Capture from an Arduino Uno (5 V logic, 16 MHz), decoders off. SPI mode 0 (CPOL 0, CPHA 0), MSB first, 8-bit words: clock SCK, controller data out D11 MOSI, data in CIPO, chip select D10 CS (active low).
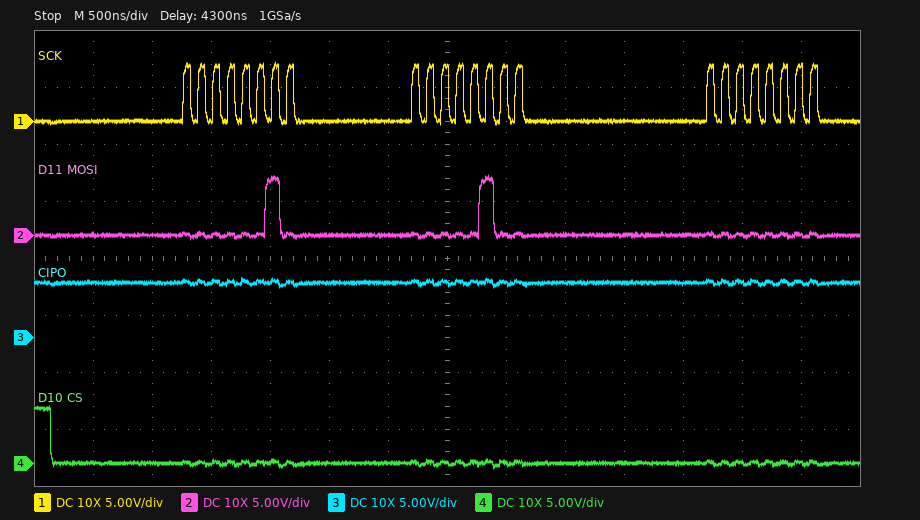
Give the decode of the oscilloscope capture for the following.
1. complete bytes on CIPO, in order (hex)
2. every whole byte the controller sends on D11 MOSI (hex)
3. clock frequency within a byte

FF FF FF
02 04 00
8 MHz
